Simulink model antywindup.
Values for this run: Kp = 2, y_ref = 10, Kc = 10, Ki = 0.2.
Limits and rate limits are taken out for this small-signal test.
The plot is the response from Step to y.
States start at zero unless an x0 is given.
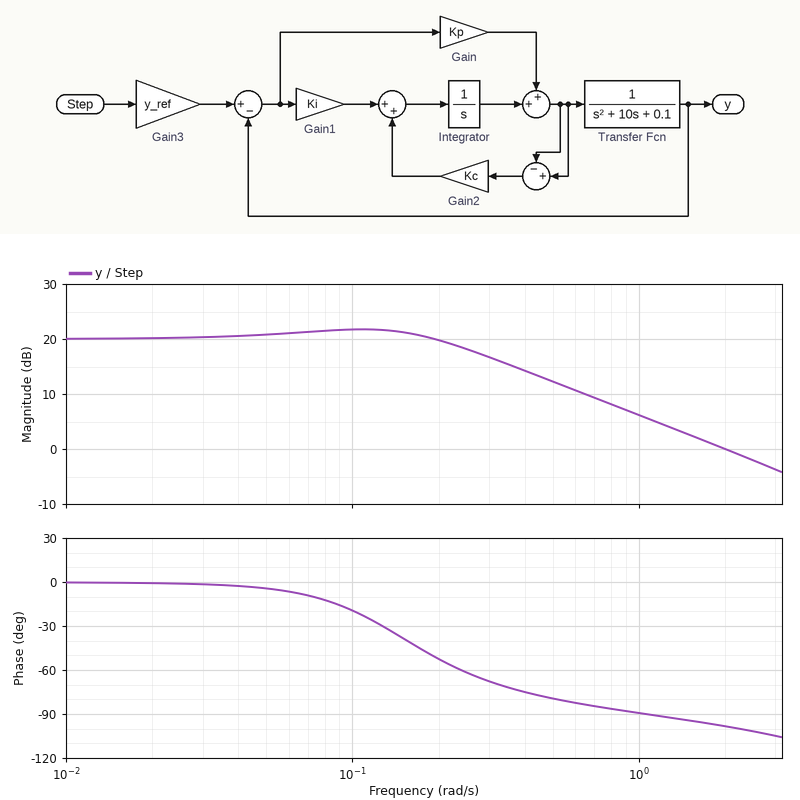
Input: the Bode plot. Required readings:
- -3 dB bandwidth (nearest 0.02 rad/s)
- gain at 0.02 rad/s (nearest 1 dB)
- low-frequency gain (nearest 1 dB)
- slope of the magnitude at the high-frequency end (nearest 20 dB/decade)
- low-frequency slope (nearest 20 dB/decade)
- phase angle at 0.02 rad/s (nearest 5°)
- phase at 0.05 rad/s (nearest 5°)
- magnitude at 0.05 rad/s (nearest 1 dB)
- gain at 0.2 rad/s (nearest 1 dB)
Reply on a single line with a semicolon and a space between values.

0.28 rad/s; 20 dB; 20 dB; -20 dB/decade; 0 dB/decade; 0°; -5°; 21 dB; 20 dB
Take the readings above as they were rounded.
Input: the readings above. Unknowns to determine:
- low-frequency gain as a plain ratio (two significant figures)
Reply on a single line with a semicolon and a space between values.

10
